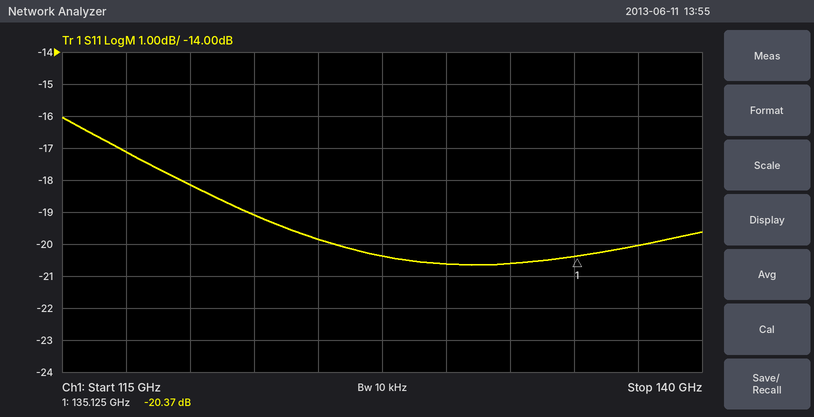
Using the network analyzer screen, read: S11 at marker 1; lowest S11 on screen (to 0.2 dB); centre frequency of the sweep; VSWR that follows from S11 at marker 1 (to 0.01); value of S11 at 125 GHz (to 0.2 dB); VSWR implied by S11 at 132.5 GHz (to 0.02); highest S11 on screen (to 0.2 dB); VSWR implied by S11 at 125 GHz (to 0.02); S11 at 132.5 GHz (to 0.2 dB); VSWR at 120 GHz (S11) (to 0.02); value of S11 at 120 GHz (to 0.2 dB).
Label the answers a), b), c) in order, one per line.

a) -20.37 dB
b) -20.6 dB
c) 127.5 GHz
d) 1.21
e) -19.8 dB
f) 1.20
g) -16.0 dB
h) 1.22
i) -20.6 dB
j) 1.28
k) -18.2 dB
